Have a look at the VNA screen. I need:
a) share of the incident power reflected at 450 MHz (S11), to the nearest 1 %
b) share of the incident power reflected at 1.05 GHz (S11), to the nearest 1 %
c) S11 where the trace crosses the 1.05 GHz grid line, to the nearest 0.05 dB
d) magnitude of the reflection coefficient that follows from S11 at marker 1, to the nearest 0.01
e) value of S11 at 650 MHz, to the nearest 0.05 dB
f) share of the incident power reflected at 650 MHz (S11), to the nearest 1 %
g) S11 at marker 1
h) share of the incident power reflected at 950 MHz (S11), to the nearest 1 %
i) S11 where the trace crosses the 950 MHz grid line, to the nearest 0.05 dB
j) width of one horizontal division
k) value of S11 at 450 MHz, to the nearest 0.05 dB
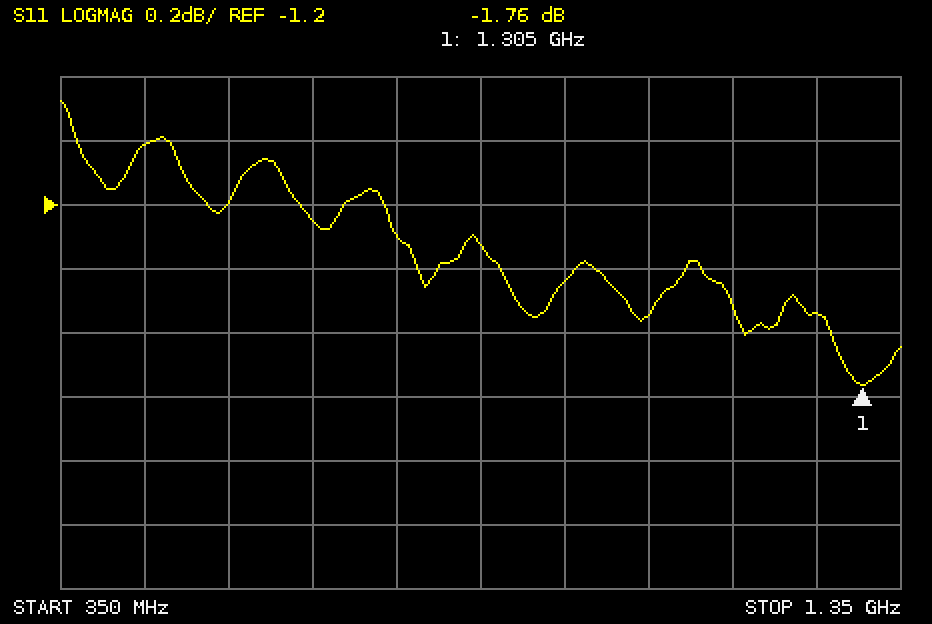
79 %
70 %
-1.55 dB
0.82
-1.25 dB
75 %
-1.76 dB
72 %
-1.45 dB
100 MHz
-1.00 dB
